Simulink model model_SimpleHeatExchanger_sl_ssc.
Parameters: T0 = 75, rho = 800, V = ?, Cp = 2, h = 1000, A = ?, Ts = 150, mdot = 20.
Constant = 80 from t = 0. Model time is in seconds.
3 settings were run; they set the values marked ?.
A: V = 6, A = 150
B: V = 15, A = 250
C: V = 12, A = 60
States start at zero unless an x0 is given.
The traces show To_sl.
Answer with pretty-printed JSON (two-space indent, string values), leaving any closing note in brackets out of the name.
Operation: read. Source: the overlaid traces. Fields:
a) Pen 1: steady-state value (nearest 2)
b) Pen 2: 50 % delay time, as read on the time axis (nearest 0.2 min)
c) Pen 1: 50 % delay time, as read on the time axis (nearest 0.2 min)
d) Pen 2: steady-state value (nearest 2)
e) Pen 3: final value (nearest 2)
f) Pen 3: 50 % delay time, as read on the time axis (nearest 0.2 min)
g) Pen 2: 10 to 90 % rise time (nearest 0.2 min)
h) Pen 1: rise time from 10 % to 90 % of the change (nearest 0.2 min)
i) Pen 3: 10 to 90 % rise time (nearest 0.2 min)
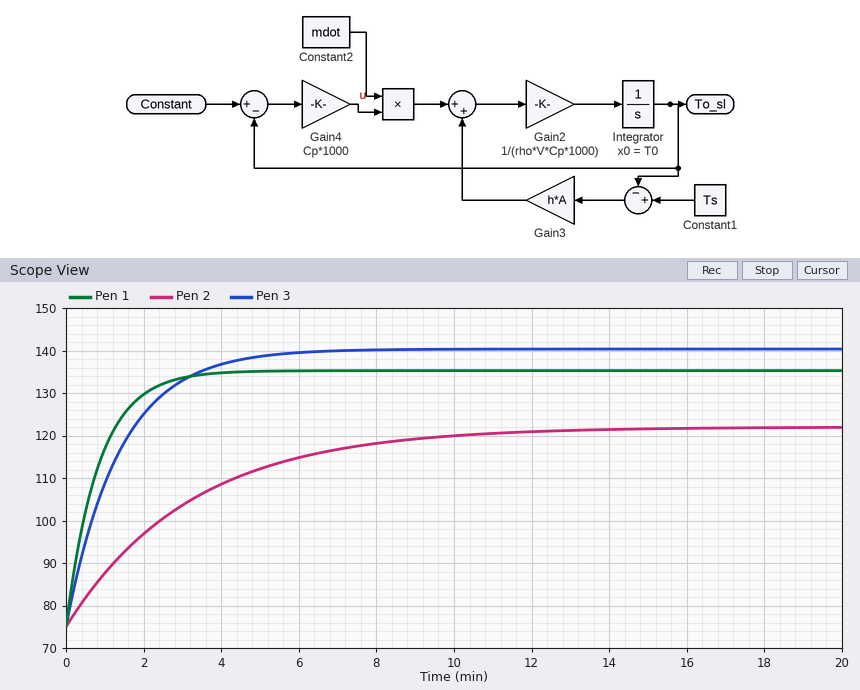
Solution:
{
  "Pen 1: steady-state value": "136",
  "Pen 2: 50 % delay time, as read on the time axis": "2.2 min",
  "Pen 1: 50 % delay time, as read on the time axis": "0.6 min",
  "Pen 2: steady-state value": "122",
  "Pen 3: final value": "140",
  "Pen 3: 50 % delay time, as read on the time axis": "1.0 min",
  "Pen 2: 10 to 90 % rise time": "7.0 min",
  "Pen 1: rise time from 10 % to 90 % of the change": "1.8 min",
  "Pen 3: 10 to 90 % rise time": "3.0 min"
}
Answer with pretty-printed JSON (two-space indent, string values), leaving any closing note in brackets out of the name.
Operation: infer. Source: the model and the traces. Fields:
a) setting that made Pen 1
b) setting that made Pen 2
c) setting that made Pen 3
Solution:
{
  "setting that made Pen 1": "A",
  "setting that made Pen 2": "C",
  "setting that made Pen 3": "B"
}
